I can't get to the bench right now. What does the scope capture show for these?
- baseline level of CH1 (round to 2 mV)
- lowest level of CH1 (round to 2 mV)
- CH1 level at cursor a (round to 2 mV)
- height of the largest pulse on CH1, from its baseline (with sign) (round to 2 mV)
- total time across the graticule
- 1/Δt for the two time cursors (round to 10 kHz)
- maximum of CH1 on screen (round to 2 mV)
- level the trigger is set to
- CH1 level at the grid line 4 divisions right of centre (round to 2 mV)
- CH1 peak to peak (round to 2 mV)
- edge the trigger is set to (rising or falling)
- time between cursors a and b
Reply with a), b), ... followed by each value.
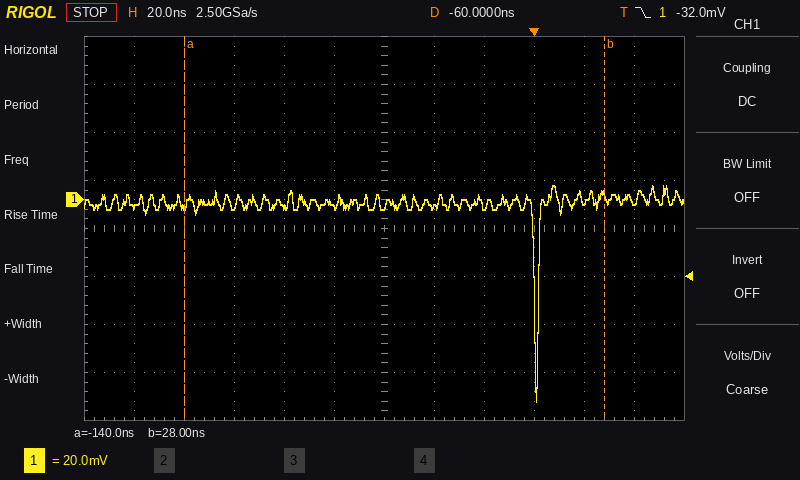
a) -2 mV
b) -84 mV
c) -2 mV
d) -82 mV
e) 240 ns
f) 5.95 MHz
g) 6 mV
h) -32.0 mV
i) 0 mV
j) 90 mV
k) falling
l) 168 ns
